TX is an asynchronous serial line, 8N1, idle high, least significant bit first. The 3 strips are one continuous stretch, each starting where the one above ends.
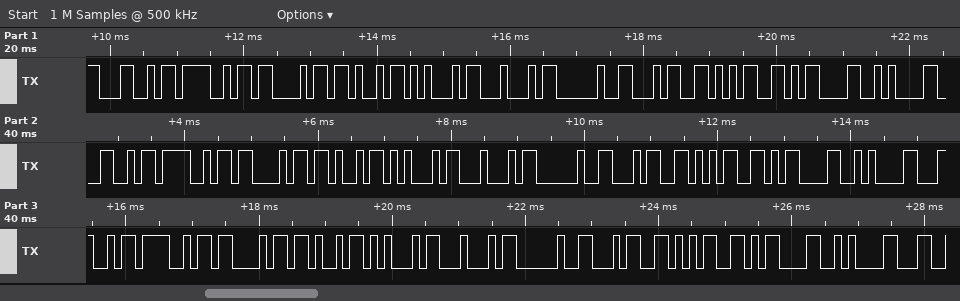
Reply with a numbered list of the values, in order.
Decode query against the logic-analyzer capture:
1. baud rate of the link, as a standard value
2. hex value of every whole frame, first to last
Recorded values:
1. 9600 baud
2. 4C 4F 43 4B 45 44 20 34 35 0D 0A 4C 4F 43 4B 45 44 20 34 35 0D 0A 4C 4F 43 4B 45 44 20 34 35 0D 0A
